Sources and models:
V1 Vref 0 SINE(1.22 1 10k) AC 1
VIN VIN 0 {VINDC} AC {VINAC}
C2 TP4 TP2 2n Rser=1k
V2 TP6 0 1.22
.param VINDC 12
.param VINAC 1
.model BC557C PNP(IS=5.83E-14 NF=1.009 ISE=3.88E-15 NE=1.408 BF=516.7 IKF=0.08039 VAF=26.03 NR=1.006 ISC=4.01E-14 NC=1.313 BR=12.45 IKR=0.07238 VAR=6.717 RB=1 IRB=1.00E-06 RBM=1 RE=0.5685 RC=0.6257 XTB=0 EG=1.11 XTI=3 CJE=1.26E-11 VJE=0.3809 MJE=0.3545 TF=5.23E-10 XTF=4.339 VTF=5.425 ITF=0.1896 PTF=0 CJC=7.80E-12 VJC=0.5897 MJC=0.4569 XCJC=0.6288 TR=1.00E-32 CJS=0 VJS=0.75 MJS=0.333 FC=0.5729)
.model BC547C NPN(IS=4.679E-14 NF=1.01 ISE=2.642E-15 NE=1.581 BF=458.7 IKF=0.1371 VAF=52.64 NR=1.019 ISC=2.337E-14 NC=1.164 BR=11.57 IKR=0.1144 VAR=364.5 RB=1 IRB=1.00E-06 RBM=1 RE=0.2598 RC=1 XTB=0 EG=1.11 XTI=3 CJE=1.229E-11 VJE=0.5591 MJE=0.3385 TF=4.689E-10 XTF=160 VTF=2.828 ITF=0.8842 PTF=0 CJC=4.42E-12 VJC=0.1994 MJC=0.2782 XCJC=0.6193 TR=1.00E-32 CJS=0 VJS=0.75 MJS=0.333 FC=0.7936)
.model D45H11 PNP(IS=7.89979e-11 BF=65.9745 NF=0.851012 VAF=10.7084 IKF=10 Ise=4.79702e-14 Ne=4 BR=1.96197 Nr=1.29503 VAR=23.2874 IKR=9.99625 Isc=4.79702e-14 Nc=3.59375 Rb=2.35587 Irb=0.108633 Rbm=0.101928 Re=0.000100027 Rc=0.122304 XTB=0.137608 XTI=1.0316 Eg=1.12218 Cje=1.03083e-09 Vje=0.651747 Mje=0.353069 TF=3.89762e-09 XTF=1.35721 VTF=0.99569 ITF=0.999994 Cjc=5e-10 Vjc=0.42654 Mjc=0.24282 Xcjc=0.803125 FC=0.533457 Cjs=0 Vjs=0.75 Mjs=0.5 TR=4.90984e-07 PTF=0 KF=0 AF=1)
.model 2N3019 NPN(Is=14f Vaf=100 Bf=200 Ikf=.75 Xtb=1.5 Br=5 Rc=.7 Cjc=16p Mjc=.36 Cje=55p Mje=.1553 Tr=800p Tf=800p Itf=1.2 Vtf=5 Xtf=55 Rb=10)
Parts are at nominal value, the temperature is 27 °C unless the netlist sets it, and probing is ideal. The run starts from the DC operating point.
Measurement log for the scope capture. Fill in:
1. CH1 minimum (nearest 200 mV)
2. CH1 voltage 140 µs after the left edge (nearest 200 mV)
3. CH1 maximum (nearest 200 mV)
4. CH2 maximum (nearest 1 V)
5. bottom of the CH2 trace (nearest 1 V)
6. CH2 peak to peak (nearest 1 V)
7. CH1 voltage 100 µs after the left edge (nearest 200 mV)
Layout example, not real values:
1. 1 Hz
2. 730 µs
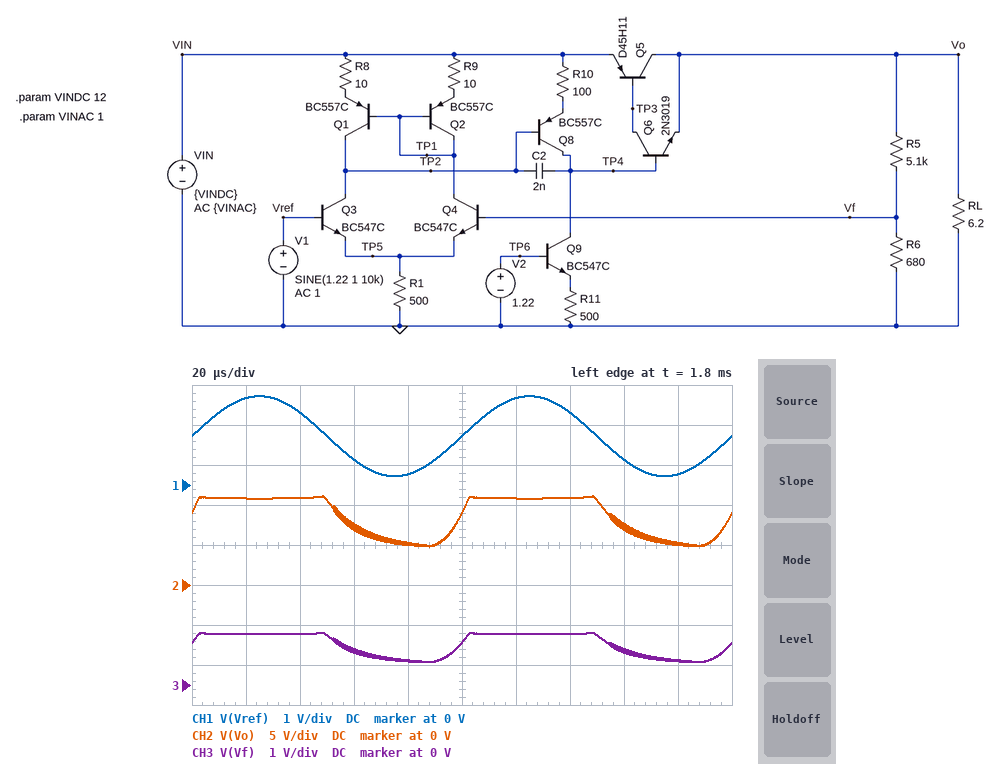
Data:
1. 200 mV
2. 1.8 V
3. 2.2 V
4. 11 V
5. 5 V
6. 6 V
7. 1.2 V
